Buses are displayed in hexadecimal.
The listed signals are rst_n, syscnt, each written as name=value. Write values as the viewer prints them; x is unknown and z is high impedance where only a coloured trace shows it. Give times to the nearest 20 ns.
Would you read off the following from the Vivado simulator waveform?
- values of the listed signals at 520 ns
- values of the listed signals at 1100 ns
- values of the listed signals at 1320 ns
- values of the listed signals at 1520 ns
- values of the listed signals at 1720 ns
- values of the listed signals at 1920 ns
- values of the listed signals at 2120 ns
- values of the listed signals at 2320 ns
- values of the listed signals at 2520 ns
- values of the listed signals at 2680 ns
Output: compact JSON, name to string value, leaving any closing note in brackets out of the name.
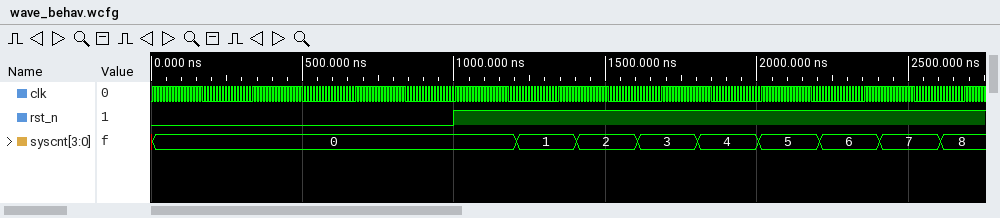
{"values of the listed signals at 520 ns": "rst_n=0, syscnt=0", "values of the listed signals at 1100 ns": "rst_n=1, syscnt=0", "values of the listed signals at 1320 ns": "rst_n=1, syscnt=1", "values of the listed signals at 1520 ns": "rst_n=1, syscnt=2", "values of the listed signals at 1720 ns": "rst_n=1, syscnt=3", "values of the listed signals at 1920 ns": "rst_n=1, syscnt=4", "values of the listed signals at 2120 ns": "rst_n=1, syscnt=5", "values of the listed signals at 2320 ns": "rst_n=1, syscnt=6", "values of the listed signals at 2520 ns": "rst_n=1, syscnt=7", "values of the listed signals at 2680 ns": "rst_n=1, syscnt=8"}
